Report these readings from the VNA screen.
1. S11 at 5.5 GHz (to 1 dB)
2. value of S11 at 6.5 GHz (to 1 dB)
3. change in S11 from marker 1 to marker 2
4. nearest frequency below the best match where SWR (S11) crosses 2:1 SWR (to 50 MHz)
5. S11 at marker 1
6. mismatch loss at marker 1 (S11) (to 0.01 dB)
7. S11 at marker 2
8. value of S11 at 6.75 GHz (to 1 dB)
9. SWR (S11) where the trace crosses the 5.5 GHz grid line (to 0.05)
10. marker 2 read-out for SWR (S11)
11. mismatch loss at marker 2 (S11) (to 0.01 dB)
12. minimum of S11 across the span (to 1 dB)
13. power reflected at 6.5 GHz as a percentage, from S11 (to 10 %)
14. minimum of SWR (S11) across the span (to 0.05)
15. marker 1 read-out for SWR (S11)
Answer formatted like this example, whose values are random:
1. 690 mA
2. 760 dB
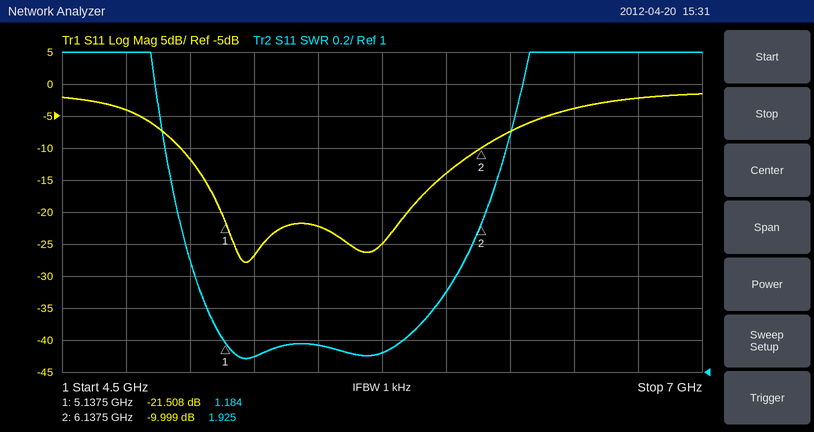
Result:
1. -22 dB
2. -4 dB
3. 11.509 dB
4. 4.95 GHz
5. -21.508 dB
6. 0.03 dB
7. -9.999 dB
8. -2 dB
9. 1.15
10. 1.925
11. 0.46 dB
12. -28 dB
13. 40 %
14. 1.10
15. 1.184
